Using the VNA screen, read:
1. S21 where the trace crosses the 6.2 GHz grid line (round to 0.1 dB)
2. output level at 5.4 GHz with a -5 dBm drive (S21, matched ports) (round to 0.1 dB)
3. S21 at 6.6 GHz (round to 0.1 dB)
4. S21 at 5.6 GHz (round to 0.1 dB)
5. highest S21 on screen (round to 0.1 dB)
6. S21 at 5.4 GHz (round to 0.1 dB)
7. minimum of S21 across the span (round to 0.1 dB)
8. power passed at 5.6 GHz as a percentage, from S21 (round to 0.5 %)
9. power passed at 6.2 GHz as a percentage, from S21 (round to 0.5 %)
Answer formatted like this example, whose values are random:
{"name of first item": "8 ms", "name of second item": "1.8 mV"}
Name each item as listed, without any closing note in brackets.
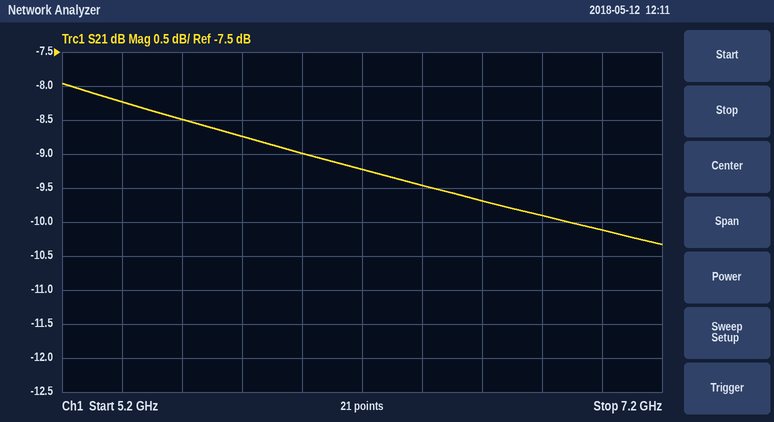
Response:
{"S21 where the trace crosses the 6.2 GHz grid line": "-9.2 dB", "output level at 5.4 GHz with a -5 dBm drive (S21, matched ports)": "-13.2 dBm", "S21 at 6.6 GHz": "-9.7 dB", "S21 at 5.6 GHz": "-8.5 dB", "highest S21 on screen": "-8.0 dB", "S21 at 5.4 GHz": "-8.2 dB", "minimum of S21 across the span": "-10.3 dB", "power passed at 5.6 GHz as a percentage, from S21": "14.0 %", "power passed at 6.2 GHz as a percentage, from S21": "12.0 %"}
